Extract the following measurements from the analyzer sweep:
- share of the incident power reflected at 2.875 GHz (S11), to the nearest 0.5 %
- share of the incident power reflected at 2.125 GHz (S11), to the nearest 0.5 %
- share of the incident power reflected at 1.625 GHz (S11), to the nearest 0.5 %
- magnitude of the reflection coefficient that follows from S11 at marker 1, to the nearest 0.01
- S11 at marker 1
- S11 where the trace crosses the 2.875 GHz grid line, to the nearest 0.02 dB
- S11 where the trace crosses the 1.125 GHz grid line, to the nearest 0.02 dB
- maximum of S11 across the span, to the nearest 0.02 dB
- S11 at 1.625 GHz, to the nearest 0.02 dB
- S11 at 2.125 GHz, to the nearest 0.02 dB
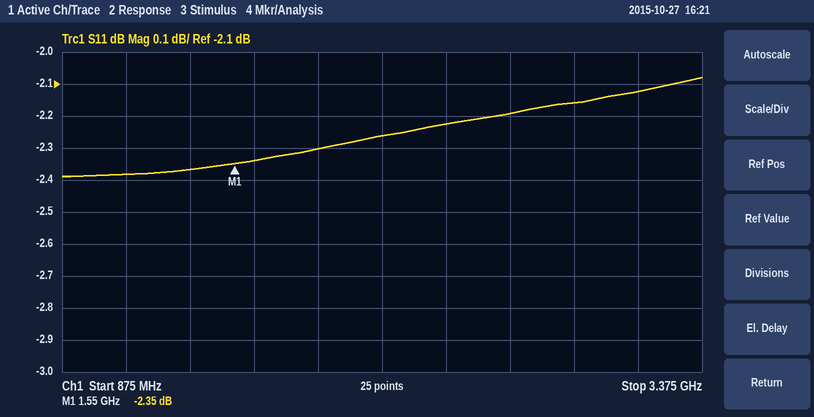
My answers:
61.0 %
59.5 %
58.5 %
0.76
-2.35 dB
-2.16 dB
-2.38 dB
-2.08 dB
-2.34 dB
-2.26 dB
